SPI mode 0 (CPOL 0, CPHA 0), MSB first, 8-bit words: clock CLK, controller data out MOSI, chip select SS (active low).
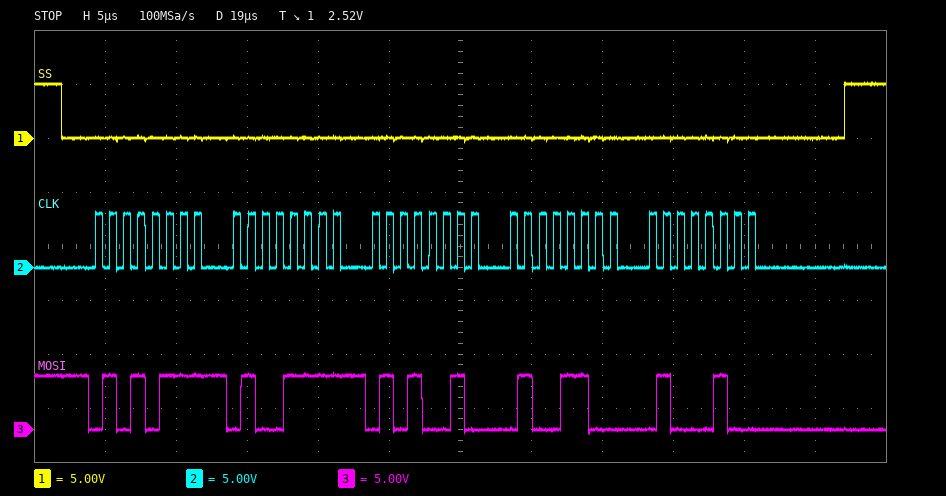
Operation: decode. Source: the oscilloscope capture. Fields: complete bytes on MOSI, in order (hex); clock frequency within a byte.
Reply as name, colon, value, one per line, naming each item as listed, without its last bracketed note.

complete bytes on MOSI, in order: 57 4F 52 4C 44
clock frequency within a byte: 1 MHz
